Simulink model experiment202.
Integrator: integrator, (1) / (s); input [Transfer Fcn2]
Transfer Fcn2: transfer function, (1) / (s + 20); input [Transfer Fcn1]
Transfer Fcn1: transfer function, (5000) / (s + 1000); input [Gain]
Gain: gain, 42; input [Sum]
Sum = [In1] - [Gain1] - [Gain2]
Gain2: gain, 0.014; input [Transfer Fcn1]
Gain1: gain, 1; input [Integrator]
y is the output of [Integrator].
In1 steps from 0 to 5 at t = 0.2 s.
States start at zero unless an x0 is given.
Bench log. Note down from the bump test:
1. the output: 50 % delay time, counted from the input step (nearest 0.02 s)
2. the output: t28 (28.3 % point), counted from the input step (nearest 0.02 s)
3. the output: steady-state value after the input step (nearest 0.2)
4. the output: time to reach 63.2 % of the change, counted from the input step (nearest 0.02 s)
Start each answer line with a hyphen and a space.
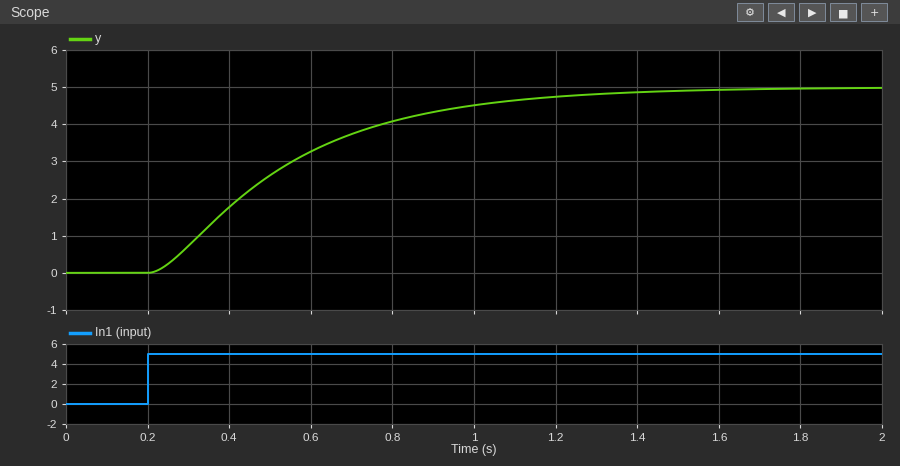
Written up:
- 0.28 s
- 0.16 s
- 5.0
- 0.38 s
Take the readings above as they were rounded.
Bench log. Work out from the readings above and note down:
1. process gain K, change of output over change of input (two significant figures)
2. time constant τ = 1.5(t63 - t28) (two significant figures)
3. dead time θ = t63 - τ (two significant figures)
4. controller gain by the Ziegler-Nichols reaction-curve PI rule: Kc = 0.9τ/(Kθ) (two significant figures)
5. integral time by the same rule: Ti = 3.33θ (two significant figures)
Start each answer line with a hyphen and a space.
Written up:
- 1.0
- 0.33 s
- 0.050 s
- 5.9
- 0.17 s
